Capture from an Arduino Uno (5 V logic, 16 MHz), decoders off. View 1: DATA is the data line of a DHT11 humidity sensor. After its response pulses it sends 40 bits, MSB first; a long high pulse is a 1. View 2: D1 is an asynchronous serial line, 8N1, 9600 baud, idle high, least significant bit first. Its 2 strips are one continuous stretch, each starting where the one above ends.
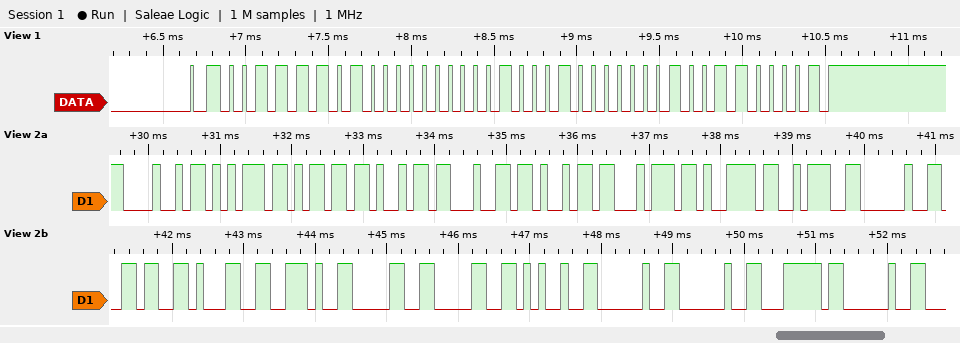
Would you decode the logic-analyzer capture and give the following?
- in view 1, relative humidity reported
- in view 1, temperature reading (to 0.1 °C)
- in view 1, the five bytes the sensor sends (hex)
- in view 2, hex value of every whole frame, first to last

61 %
34.2 °C
3D 00 22 02 61
0x48 0x75 0x6D 0x69 0x64 0x69 0x74 0x79 0x3A 0x20 0x36 0x31 0x2E 0x30 0x30 0x25 0x20 0x20 0x7C 0x20
